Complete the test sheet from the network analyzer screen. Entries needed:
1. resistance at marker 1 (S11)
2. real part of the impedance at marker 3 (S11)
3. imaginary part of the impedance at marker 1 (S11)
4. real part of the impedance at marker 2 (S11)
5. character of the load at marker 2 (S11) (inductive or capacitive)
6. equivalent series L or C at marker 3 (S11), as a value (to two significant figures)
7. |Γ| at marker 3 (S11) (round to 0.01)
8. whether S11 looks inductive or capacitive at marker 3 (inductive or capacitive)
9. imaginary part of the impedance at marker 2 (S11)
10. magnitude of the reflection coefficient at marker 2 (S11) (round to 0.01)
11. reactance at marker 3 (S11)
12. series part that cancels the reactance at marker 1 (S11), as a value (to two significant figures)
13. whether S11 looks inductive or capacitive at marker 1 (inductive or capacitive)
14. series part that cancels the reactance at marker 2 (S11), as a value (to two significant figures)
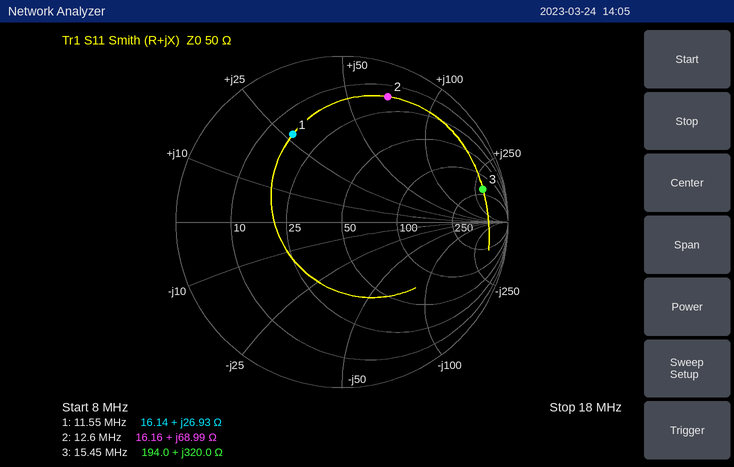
16.14 Ω
194.0 Ω
+26.93 Ω
16.16 Ω
inductive
3.3 µH
0.87
inductive
+68.99 Ω
0.80
+320.0 Ω
510 pF
inductive
180 pF
